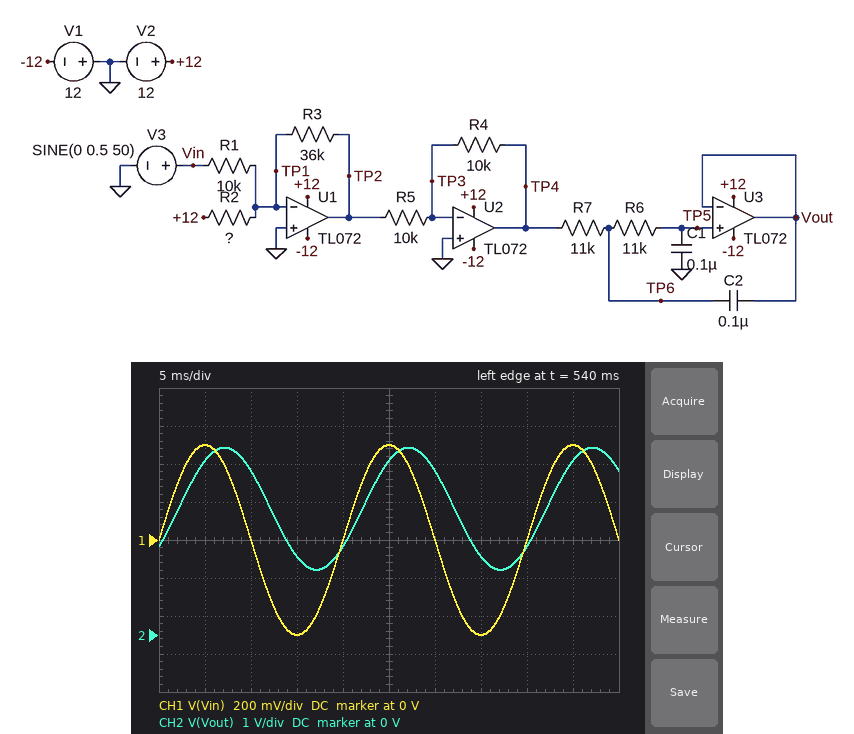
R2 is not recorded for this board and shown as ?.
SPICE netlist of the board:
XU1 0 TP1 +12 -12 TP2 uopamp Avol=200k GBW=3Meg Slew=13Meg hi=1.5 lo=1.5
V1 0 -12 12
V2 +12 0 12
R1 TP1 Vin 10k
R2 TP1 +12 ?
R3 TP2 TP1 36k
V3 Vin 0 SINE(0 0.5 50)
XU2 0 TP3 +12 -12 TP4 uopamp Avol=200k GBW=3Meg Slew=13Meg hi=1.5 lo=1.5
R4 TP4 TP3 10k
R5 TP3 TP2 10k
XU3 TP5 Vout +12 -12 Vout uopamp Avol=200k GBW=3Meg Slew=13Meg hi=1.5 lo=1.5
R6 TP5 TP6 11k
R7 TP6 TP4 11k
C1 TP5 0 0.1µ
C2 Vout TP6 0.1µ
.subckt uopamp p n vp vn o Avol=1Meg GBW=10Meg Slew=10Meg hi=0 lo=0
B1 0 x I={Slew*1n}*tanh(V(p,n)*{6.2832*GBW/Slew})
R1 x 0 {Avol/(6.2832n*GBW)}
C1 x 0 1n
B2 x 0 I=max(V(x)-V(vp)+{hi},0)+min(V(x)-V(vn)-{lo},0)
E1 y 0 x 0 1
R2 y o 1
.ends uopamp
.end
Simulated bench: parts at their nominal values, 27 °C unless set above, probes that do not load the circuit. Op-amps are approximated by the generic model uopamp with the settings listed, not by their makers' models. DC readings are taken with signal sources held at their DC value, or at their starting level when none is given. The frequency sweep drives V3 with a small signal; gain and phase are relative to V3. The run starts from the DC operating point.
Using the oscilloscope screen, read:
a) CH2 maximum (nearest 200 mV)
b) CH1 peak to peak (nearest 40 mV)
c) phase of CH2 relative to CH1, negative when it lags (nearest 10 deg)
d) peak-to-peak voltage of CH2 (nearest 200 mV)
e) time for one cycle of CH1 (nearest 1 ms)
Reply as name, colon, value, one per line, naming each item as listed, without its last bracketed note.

CH2 maximum: 5.0 V
CH1 peak to peak: 1.00 V
phase of CH2 relative to CH1, negative when it lags: -40 deg
peak-to-peak voltage of CH2: 3.2 V
time for one cycle of CH1: 20 ms
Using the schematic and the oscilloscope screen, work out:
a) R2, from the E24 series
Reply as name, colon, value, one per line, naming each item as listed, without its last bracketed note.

R2, from the E24 series: 130 kΩ
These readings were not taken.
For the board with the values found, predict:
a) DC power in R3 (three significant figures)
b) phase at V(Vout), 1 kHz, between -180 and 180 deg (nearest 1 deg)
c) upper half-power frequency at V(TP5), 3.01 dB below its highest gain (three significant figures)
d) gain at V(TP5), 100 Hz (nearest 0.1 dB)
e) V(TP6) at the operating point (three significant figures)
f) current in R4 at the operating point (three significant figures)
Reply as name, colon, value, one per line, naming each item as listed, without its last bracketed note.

DC power in R3: 307 µW
phase at V(Vout), 1 kHz, between -180 and 180 deg: -164 deg
upper half-power frequency at V(TP5), 3.01 dB below its highest gain: 93.1 Hz
gain at V(TP5), 100 Hz: 7.7 dB
V(TP6) at the operating point: 3.32 V
current in R4 at the operating point: 332 µA
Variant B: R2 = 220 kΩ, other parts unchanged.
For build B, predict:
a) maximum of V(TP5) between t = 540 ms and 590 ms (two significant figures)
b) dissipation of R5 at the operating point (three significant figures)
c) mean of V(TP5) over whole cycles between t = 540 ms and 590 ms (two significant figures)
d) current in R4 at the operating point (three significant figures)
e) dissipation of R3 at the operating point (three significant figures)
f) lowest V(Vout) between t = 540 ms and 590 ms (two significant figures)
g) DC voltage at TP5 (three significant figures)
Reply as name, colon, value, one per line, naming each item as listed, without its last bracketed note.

maximum of V(TP5) between t = 540 ms and 590 ms: 3.6 V
dissipation of R5 at the operating point: 386 µW
mean of V(TP5) over whole cycles between t = 540 ms and 590 ms: 2.0 V
current in R4 at the operating point: 196 µA
dissipation of R3 at the operating point: 107 µW
lowest V(Vout) between t = 540 ms and 590 ms: 360 mV
DC voltage at TP5: 1.96 V
